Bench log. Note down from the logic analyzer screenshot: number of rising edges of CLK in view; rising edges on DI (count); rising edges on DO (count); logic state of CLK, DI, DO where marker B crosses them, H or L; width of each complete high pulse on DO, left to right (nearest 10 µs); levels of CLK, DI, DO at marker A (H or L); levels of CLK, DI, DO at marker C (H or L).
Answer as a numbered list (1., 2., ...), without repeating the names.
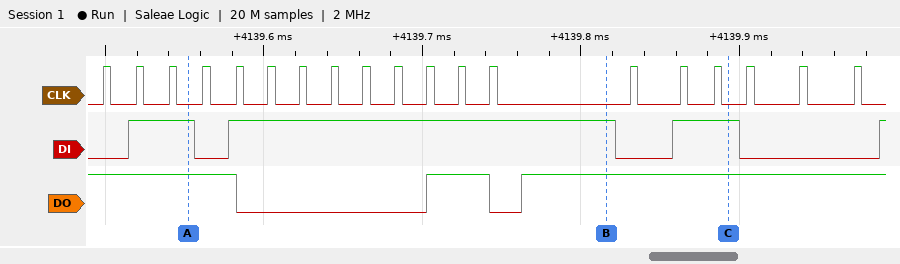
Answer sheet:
1. 19
2. 4
3. 2
4. CLK=L, DI=H, DO=H
5. 40 µs
6. CLK=L, DI=H, DO=H
7. CLK=L, DI=H, DO=H
